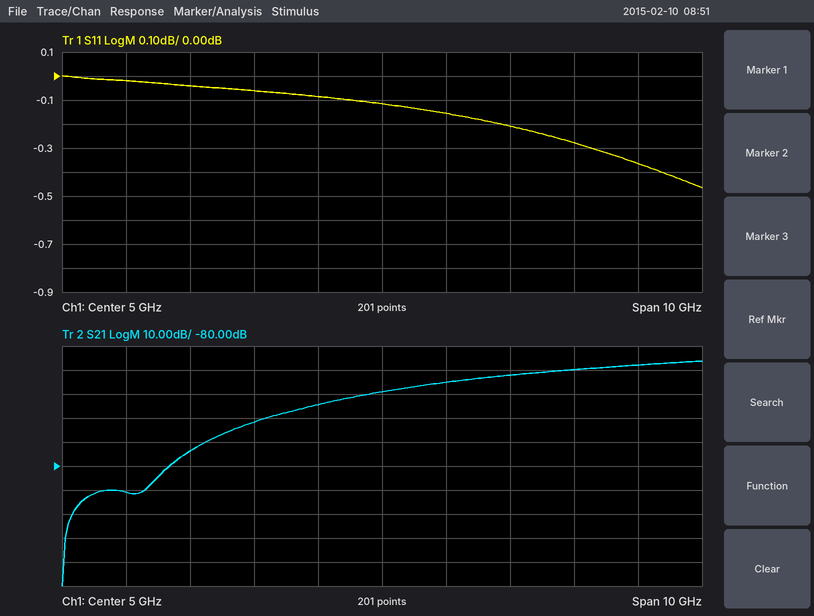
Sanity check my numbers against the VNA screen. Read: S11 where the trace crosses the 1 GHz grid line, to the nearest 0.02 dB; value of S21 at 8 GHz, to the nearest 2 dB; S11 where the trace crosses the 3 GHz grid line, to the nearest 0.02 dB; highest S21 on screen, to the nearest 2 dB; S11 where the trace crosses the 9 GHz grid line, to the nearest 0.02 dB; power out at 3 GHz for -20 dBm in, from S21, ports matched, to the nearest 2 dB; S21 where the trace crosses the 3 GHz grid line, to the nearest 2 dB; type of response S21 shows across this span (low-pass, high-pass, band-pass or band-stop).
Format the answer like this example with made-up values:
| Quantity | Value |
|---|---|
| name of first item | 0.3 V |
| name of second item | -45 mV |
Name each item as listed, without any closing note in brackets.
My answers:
| Quantity | Value |
|---|---|
| S11 where the trace crosses the 1 GHz grid line, to the nearest 0.02 dB | -0.02 dB |
| value of S21 at 8 GHz, to the nearest 2 dB | -40 dB |
| S11 where the trace crosses the 3 GHz grid line, to the nearest 0.02 dB | -0.06 dB |
| highest S21 on screen, to the nearest 2 dB | -36 dB |
| S11 where the trace crosses the 9 GHz grid line, to the nearest 0.02 dB | -0.36 dB |
| power out at 3 GHz for -20 dBm in, from S21, ports matched, to the nearest 2 dB | -82 dBm |
| S21 where the trace crosses the 3 GHz grid line, to the nearest 2 dB | -62 dB |
| type of response S21 shows across this span | high-pass |
